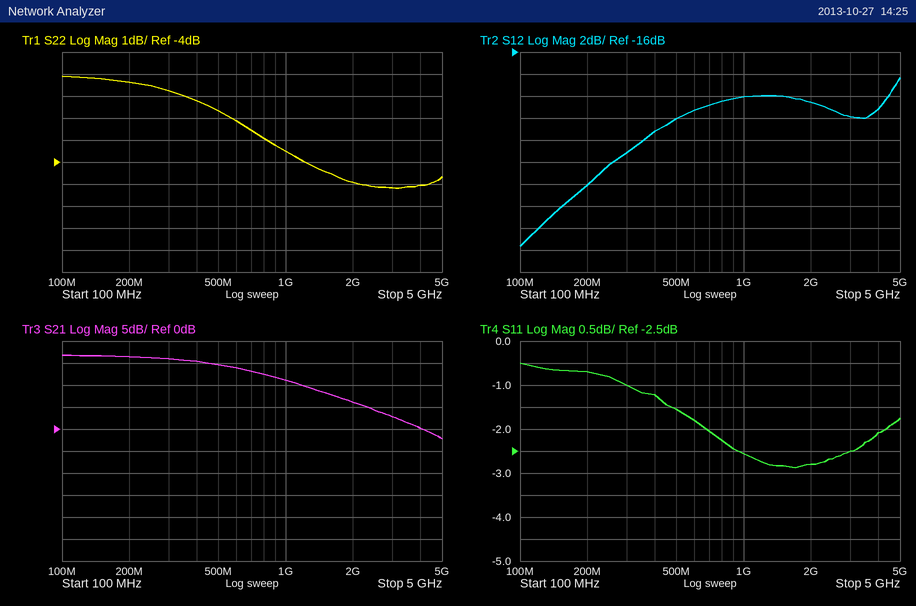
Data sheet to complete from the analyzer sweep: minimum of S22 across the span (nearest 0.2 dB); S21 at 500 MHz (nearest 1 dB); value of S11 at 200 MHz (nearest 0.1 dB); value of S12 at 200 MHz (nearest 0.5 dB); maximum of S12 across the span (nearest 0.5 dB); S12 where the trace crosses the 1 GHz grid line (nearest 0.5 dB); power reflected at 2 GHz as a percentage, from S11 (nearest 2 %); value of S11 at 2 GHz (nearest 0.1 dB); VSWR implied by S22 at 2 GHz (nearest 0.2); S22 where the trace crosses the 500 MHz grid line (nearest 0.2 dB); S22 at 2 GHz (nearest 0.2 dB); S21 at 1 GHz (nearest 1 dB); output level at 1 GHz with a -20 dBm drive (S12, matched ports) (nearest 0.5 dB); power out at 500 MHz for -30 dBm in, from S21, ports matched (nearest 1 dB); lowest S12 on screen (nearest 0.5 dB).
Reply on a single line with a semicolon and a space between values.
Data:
-5.2 dB; 15 dB; -0.7 dB; -28.0 dB; -18.5 dB; -20.0 dB; 52 %; -2.8 dB; 3.6; -1.6 dB; -5.0 dB; 11 dB; -40.0 dBm; -15 dBm; -33.5 dB
